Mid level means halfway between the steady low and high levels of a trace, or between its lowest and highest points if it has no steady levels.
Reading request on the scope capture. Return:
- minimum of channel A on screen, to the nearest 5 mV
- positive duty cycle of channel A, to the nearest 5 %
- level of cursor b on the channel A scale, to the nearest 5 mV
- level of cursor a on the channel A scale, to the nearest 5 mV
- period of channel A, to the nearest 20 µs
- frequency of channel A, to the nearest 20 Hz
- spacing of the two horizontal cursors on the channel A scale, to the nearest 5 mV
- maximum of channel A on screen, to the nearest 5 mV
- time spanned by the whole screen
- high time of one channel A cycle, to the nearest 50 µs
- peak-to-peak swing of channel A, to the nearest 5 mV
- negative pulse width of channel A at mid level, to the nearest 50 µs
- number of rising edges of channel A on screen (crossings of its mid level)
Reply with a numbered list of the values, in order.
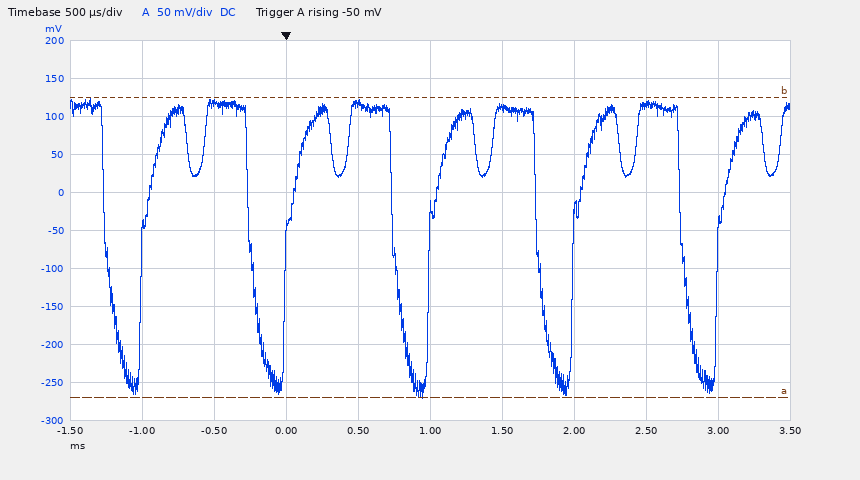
1. -270 mV
2. 75 %
3. 125 mV
4. -270 mV
5. 1.00 ms
6. 1.00 kHz
7. 395 mV
8. 125 mV
9. 5 ms
10. 750 µs
11. 395 mV
12. 250 µs
13. 5
